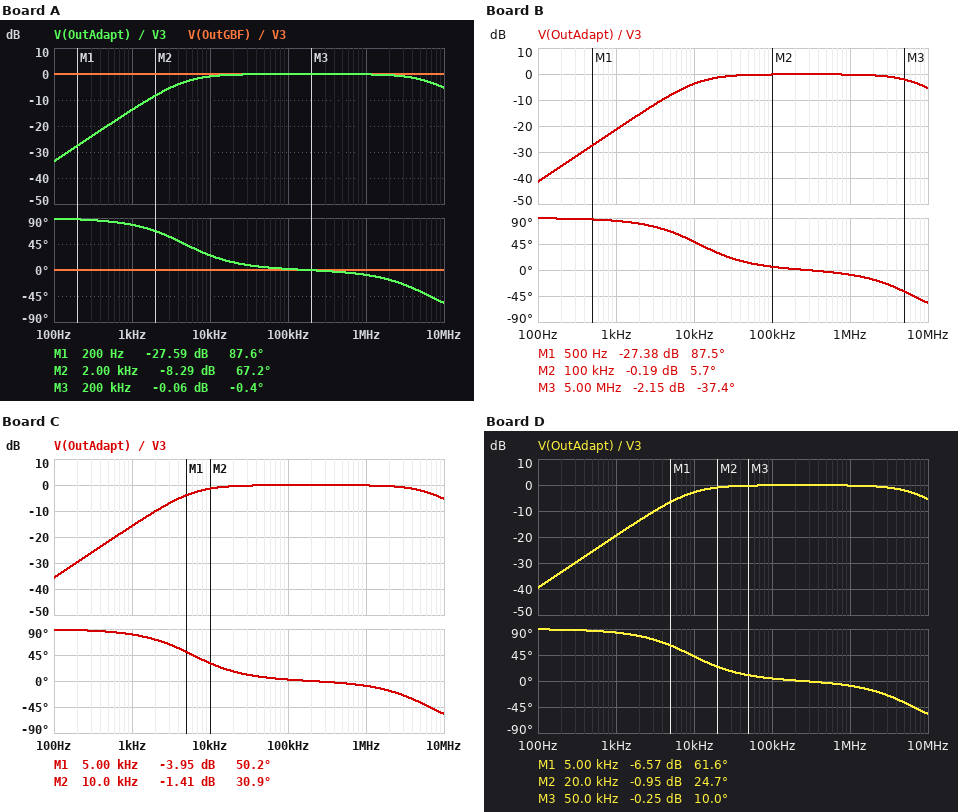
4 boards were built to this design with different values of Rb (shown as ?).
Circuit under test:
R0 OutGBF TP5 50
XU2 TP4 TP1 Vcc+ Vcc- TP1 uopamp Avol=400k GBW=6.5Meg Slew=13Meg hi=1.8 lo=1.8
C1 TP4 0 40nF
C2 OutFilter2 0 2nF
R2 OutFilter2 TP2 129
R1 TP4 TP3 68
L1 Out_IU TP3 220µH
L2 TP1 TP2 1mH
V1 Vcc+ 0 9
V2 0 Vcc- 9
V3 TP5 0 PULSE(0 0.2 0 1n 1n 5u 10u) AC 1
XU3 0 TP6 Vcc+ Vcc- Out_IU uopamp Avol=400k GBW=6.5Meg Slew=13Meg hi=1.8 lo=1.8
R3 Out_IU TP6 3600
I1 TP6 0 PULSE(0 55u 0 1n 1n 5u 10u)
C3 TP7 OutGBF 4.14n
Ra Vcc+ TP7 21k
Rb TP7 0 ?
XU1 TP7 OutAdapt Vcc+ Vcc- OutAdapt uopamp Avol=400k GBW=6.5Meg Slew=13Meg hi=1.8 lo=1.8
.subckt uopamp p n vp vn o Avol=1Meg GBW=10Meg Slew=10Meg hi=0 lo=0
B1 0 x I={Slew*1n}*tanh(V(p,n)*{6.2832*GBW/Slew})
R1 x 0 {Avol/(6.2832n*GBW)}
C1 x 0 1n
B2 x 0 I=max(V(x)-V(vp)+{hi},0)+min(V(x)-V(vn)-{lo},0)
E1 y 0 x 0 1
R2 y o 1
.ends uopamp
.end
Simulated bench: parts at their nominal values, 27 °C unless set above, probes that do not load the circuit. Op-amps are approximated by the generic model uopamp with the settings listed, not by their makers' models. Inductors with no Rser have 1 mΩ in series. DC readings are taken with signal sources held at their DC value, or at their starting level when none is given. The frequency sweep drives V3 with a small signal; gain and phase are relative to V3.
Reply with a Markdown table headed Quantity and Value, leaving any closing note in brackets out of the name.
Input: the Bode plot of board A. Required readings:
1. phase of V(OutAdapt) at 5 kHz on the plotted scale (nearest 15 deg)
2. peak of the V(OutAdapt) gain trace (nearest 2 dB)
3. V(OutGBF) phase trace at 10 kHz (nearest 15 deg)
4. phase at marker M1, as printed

| Quantity | Value |
|---|---|
| phase of V(OutAdapt) at 5 kHz on the plotted scale | 45 deg |
| peak of the V(OutAdapt) gain trace | 0 dB |
| V(OutGBF) phase trace at 10 kHz | 0 deg |
| phase at marker M1, as printed | 87.6 deg |
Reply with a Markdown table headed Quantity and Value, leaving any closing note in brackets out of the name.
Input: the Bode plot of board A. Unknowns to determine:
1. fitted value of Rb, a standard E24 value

| Quantity | Value |
|---|---|
| fitted value of Rb, a standard E24 value | 13 kΩ |
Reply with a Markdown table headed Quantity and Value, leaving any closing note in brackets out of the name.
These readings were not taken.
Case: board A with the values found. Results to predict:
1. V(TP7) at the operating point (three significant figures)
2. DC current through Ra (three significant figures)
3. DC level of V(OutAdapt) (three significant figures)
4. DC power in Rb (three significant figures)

| Quantity | Value |
|---|---|
| V(TP7) at the operating point | 3.44 V |
| DC current through Ra | 265 µA |
| DC level of V(OutAdapt) | 3.44 V |
| DC power in Rb | 911 µW |
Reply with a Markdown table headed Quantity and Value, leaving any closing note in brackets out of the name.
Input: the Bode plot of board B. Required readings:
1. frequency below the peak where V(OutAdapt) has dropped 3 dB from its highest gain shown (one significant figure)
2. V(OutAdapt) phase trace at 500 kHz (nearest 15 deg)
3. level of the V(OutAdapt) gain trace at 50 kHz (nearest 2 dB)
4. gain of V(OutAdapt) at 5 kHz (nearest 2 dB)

| Quantity | Value |
|---|---|
| frequency below the peak where V(OutAdapt) has dropped 3 dB from its highest gain shown | 10 kHz |
| V(OutAdapt) phase trace at 500 kHz | 0 deg |
| level of the V(OutAdapt) gain trace at 50 kHz | 0 dB |
| gain of V(OutAdapt) at 5 kHz | -8 dB |
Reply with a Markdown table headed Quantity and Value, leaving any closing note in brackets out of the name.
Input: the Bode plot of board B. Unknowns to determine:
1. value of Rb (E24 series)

| Quantity | Value |
|---|---|
| value of Rb | 3.9 kΩ |
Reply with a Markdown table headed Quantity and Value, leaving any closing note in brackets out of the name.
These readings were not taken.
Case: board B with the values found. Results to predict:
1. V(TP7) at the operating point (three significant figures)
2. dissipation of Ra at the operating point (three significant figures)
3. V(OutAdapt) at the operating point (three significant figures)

| Quantity | Value |
|---|---|
| V(TP7) at the operating point | 1.41 V |
| dissipation of Ra at the operating point | 2.74 mW |
| V(OutAdapt) at the operating point | 1.41 V |
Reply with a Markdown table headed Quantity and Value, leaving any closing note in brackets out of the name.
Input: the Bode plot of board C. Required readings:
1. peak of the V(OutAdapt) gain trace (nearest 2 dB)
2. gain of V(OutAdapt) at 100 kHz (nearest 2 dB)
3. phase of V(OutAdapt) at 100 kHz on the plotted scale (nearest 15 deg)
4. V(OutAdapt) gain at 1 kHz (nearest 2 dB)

| Quantity | Value |
|---|---|
| peak of the V(OutAdapt) gain trace | 0 dB |
| gain of V(OutAdapt) at 100 kHz | 0 dB |
| phase of V(OutAdapt) at 100 kHz on the plotted scale | 0 deg |
| V(OutAdapt) gain at 1 kHz | -16 dB |
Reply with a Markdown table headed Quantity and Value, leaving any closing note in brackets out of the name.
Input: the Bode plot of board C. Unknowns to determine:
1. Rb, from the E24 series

| Quantity | Value |
|---|---|
| Rb, from the E24 series | 9.1 kΩ |
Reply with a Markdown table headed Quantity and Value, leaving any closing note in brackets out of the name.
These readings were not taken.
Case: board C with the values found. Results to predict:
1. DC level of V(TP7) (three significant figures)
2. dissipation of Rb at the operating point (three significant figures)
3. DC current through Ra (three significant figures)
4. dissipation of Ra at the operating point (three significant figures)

| Quantity | Value |
|---|---|
| DC level of V(TP7) | 2.72 V |
| dissipation of Rb at the operating point | 814 µW |
| DC current through Ra | 299 µA |
| dissipation of Ra at the operating point | 1.88 mW |
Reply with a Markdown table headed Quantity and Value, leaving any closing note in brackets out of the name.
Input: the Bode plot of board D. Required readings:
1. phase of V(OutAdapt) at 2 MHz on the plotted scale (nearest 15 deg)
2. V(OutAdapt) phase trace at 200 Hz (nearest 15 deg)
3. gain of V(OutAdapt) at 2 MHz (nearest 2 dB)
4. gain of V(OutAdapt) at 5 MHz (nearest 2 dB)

| Quantity | Value |
|---|---|
| phase of V(OutAdapt) at 2 MHz on the plotted scale | -15 deg |
| V(OutAdapt) phase trace at 200 Hz | 90 deg |
| gain of V(OutAdapt) at 2 MHz | 0 dB |
| gain of V(OutAdapt) at 5 MHz | -2 dB |
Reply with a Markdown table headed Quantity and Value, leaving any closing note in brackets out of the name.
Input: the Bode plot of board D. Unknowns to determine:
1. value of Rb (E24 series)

| Quantity | Value |
|---|---|
| value of Rb | 5.1 kΩ |
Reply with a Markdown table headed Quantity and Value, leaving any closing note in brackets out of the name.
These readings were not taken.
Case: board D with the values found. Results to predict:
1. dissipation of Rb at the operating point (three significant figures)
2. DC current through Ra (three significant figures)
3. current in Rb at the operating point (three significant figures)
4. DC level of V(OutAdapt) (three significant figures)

| Quantity | Value |
|---|---|
| dissipation of Rb at the operating point | 606 µW |
| DC current through Ra | 345 µA |
| current in Rb at the operating point | 345 µA |
| DC level of V(OutAdapt) | 1.76 V |
